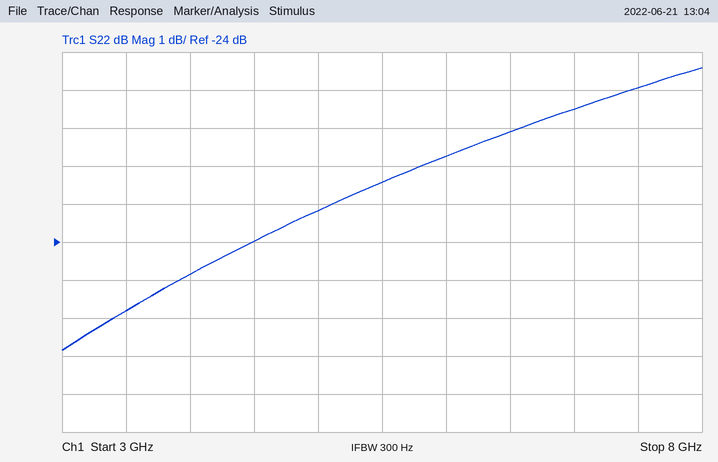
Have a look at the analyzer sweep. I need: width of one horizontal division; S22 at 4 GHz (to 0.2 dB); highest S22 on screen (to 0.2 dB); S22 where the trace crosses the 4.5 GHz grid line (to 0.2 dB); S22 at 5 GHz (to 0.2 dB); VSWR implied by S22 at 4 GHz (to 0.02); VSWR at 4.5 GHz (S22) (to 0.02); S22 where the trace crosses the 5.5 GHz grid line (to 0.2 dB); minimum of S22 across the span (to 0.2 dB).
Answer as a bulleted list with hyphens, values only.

- 500 MHz
- -24.8 dB
- -19.4 dB
- -24.0 dB
- -23.2 dB
- 1.12
- 1.14
- -22.4 dB
- -26.8 dB
